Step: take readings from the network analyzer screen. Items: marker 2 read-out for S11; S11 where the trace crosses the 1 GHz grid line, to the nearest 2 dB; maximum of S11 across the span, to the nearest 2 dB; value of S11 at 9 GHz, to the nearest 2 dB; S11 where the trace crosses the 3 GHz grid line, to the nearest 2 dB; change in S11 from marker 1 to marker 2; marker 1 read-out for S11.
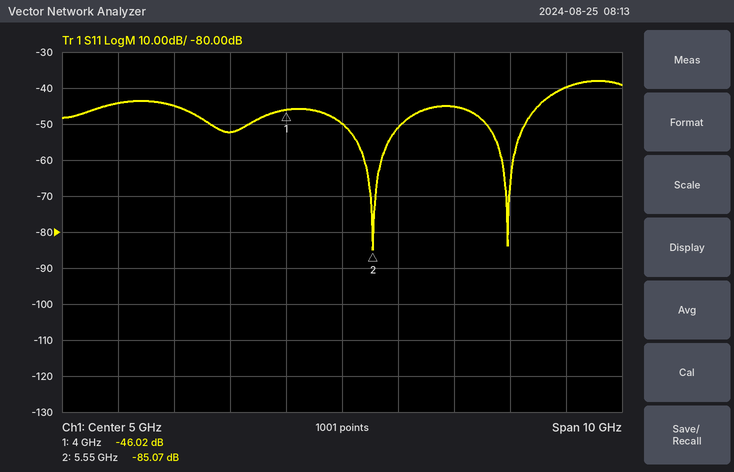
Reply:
-85.07 dB
-44 dB
-38 dB
-40 dB
-52 dB
-39.05 dB
-46.02 dB
